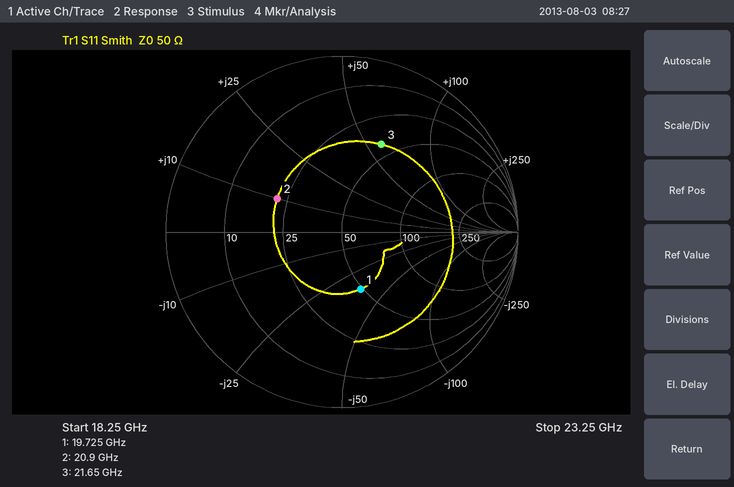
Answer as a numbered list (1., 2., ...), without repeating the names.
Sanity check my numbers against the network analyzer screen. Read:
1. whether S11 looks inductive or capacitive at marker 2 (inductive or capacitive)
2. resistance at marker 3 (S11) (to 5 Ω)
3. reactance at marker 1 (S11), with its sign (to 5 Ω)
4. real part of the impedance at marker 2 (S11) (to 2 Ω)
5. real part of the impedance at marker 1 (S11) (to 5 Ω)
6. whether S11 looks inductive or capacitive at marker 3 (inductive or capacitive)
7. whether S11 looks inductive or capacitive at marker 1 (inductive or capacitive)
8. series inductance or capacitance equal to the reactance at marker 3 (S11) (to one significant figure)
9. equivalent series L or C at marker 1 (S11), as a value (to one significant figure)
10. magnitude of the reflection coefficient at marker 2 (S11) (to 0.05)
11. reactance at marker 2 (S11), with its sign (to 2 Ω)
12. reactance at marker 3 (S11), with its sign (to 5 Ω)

1. inductive
2. 40 Ω
3. -35 Ω
4. 22 Ω
5. 50 Ω
6. inductive
7. capacitive
8. 400 pH
9. 200 fF
10. 0.40
11. +10 Ω
12. +60 Ω
